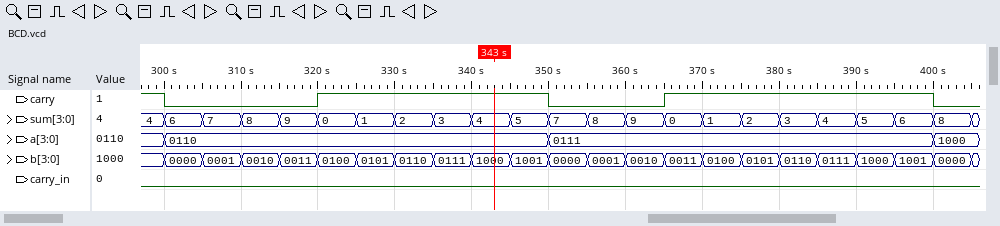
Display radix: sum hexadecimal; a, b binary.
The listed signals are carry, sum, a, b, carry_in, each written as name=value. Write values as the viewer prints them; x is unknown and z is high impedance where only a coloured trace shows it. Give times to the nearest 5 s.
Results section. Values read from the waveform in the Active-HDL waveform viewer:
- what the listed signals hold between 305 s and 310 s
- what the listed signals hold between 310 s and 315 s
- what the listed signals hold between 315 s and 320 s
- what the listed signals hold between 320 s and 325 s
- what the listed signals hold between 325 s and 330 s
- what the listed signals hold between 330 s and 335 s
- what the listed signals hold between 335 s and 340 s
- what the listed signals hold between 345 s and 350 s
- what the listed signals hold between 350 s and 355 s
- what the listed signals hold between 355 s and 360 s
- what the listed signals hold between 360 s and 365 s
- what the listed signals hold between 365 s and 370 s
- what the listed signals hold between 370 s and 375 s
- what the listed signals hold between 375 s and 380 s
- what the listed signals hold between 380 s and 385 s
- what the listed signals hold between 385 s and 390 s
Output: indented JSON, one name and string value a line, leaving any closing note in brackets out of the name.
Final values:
{
  "what the listed signals hold between 305 s and 310 s": "carry=0, sum=7, a=0110, b=0001, carry_in=0",
  "what the listed signals hold between 310 s and 315 s": "carry=0, sum=8, a=0110, b=0010, carry_in=0",
  "what the listed signals hold between 315 s and 320 s": "carry=0, sum=9, a=0110, b=0011, carry_in=0",
  "what the listed signals hold between 320 s and 325 s": "carry=1, sum=0, a=0110, b=0100, carry_in=0",
  "what the listed signals hold between 325 s and 330 s": "carry=1, sum=1, a=0110, b=0101, carry_in=0",
  "what the listed signals hold between 330 s and 335 s": "carry=1, sum=2, a=0110, b=0110, carry_in=0",
  "what the listed signals hold between 335 s and 340 s": "carry=1, sum=3, a=0110, b=0111, carry_in=0",
  "what the listed signals hold between 345 s and 350 s": "carry=1, sum=5, a=0110, b=1001, carry_in=0",
  "what the listed signals hold between 350 s and 355 s": "carry=0, sum=7, a=0111, b=0000, carry_in=0",
  "what the listed signals hold between 355 s and 360 s": "carry=0, sum=8, a=0111, b=0001, carry_in=0",
  "what the listed signals hold between 360 s and 365 s": "carry=0, sum=9, a=0111, b=0010, carry_in=0",
  "what the listed signals hold between 365 s and 370 s": "carry=1, sum=0, a=0111, b=0011, carry_in=0",
  "what the listed signals hold between 370 s and 375 s": "carry=1, sum=1, a=0111, b=0100, carry_in=0",
  "what the listed signals hold between 375 s and 380 s": "carry=1, sum=2, a=0111, b=0101, carry_in=0",
  "what the listed signals hold between 380 s and 385 s": "carry=1, sum=3, a=0111, b=0110, carry_in=0",
  "what the listed signals hold between 385 s and 390 s": "carry=1, sum=4, a=0111, b=0111, carry_in=0"
}
